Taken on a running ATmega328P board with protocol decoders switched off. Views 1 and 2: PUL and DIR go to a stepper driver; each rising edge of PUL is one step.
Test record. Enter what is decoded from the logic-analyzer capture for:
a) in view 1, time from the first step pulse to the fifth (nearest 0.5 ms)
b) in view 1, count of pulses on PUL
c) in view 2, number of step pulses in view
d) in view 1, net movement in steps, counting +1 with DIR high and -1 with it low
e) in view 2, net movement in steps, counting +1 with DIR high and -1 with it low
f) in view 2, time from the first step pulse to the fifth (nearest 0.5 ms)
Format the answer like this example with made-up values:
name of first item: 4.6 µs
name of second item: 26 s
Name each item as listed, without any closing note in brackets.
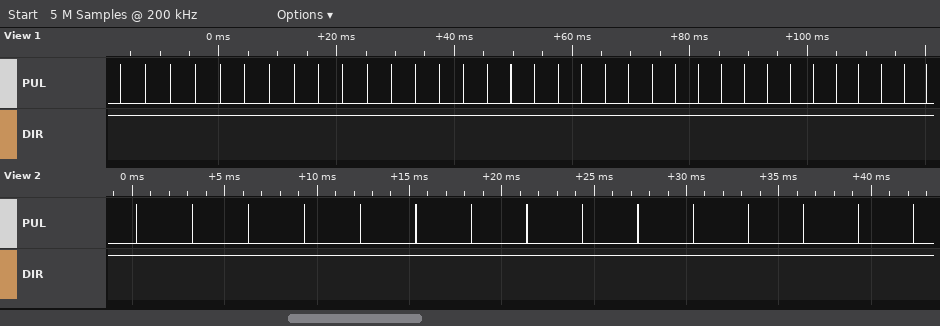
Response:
in view 1, time from the first step pulse to the fifth: 17.0 ms
in view 1, count of pulses on PUL: 35
in view 2, number of step pulses in view: 15
in view 1, net movement in steps, counting +1 with DIR high and -1 with it low: +35
in view 2, net movement in steps, counting +1 with DIR high and -1 with it low: +15
in view 2, time from the first step pulse to the fifth: 12.0 ms
